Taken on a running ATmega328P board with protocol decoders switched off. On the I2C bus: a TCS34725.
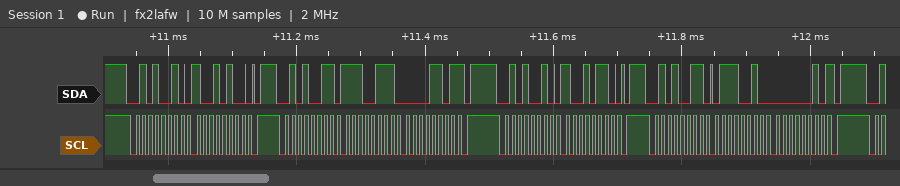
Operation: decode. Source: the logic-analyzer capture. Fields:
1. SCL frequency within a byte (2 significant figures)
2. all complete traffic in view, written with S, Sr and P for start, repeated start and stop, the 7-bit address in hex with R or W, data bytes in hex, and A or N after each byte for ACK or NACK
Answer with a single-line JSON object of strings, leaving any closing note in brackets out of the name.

{"SCL frequency within a byte": "100 kHz", "all complete traffic in view, written with S, Sr and P for start, repeated start and stop, the 7-bit address in hex with R or W, data bytes in hex, and A or N after each byte for ACK or NACK": "S 29W A 94 A P S 29R A E7 A 0D N P S 29W A 96 A P S 29R A 72 A 02 N P"}
